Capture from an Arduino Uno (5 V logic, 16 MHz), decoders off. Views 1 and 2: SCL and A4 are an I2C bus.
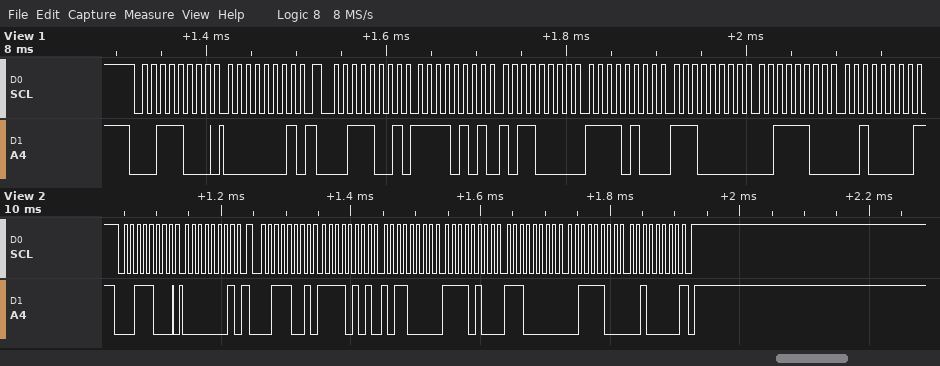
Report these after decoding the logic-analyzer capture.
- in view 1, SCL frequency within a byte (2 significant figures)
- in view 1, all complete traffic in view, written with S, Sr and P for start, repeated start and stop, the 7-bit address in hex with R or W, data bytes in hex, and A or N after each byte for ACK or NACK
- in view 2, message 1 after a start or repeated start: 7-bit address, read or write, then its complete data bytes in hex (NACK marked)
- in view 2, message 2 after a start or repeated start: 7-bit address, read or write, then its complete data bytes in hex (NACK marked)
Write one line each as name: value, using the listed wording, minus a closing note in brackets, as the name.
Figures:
in view 1, SCL frequency within a byte: 100 kHz
in view 1, all complete traffic in view, written with S, Sr and P for start, repeated start and stop, the 7-bit address in hex with R or W, data bytes in hex, and A or N after each byte for ACK or NACK: S 1CW A 01 A Sr 1CR A F5 A B0 A F4 A E0 A 3C A 20 N
in view 2, message 1 after a start or repeated start: 7-bit address, read or write, then its complete data bytes in hex: 0x1C write: 01
in view 2, message 2 after a start or repeated start: 7-bit address, read or write, then its complete data bytes in hex: 0x1C read: F5 B0 F4 E0 3C 20 NACK
